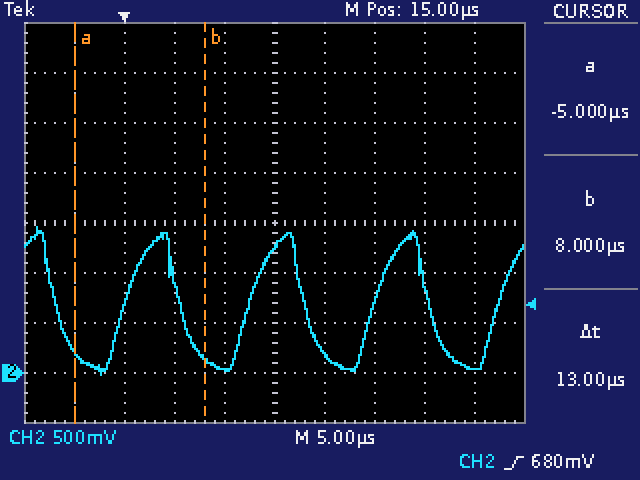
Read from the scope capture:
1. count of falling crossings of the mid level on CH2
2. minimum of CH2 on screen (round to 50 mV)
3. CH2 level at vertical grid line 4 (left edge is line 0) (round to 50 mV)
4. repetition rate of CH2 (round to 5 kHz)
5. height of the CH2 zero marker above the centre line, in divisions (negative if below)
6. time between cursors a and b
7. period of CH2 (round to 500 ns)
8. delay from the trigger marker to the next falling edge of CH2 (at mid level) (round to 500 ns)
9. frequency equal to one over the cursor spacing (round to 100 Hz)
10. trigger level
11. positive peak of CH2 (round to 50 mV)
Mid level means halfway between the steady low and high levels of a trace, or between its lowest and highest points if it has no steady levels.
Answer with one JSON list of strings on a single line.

["4", "0 mV", "50 mV", "80 kHz", "-3.0 div", "13 µs", "12.5 µs", "5.5 µs", "76.9 kHz", "680 mV", "1.45 V"]
